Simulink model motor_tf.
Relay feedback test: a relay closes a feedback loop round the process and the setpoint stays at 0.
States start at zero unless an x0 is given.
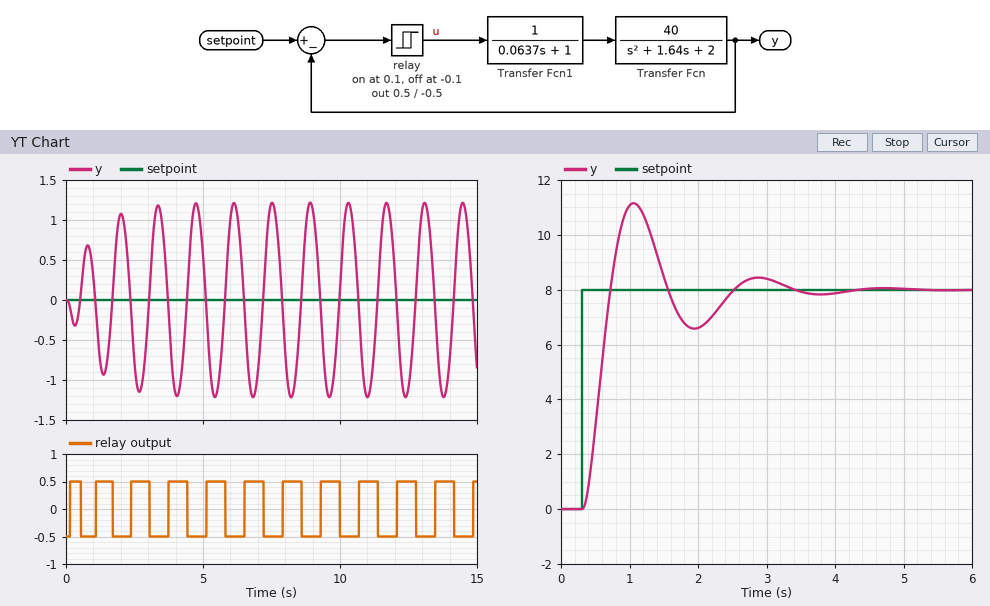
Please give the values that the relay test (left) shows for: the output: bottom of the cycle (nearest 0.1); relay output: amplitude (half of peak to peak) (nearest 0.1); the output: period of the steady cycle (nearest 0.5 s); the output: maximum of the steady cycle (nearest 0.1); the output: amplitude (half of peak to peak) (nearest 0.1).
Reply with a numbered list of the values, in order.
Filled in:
1. -1.2
2. 0.5
3. 1.5 s
4. 1.2
5. 1.2
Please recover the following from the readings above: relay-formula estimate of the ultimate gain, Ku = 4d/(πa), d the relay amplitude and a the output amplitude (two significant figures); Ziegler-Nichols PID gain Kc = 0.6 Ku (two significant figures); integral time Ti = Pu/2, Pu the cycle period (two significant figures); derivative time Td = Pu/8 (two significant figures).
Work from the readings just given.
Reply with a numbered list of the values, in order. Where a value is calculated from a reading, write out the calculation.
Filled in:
1. 4 × 0.5 / (π × 1.2) = 0.53
2. 0.6 × 0.53 = 0.32
3. 1.5 / 2 = 0.75 s
4. 1.5 / 8 = 0.19 s
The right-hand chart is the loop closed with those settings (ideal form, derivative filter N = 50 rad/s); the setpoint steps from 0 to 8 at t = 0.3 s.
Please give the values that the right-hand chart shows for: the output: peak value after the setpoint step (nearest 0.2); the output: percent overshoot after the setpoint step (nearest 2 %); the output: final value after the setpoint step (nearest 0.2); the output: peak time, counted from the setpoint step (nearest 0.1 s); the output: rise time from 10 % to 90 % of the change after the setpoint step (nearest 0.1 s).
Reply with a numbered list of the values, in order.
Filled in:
1. 11.2
2. 40 %
3. 8.0
4. 0.8 s
5. 0.3 s
